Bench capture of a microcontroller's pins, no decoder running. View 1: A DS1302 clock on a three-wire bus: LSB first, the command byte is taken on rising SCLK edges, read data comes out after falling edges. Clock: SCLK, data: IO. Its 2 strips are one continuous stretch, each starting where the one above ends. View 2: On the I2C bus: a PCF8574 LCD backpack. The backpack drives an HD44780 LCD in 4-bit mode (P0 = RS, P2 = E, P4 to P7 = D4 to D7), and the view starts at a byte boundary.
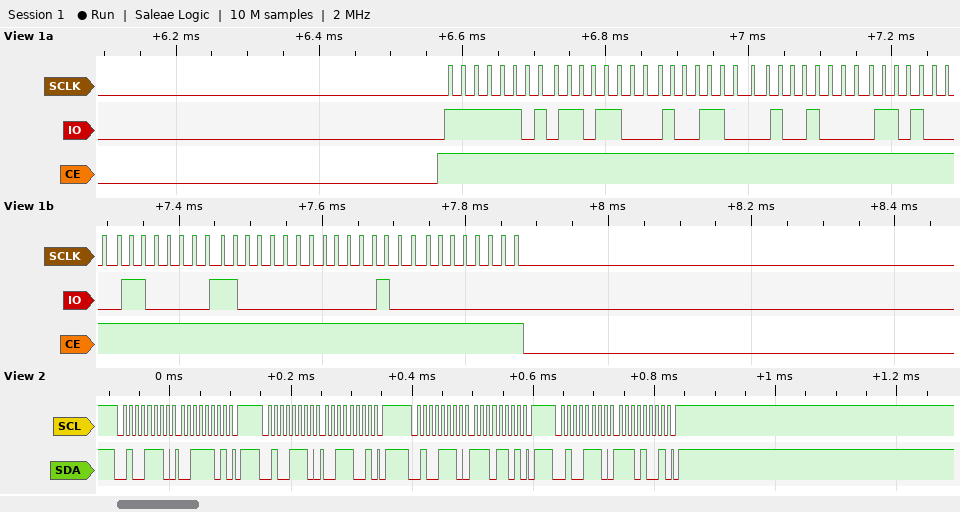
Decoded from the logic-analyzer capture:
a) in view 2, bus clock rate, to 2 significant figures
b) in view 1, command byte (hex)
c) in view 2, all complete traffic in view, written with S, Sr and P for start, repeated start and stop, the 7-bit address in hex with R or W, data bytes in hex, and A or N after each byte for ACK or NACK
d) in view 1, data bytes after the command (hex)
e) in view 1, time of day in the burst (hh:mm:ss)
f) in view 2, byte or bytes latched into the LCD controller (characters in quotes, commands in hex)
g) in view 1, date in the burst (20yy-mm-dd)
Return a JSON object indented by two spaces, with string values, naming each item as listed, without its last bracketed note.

{
  "in view 2, bus clock rate, to 2 significant figures": "100 kHz",
  "in view 1, command byte": "0xBF",
  "in view 2, all complete traffic in view, written with S, Sr and P for start, repeated start and stop, the 7-bit address in hex with R or W, data bytes in hex, and A or N after each byte for ACK or NACK": "S 27W A 3D A P S 27W A 39 A P S 27W A ED A P S 27W A E9 A P",
  "in view 1, data bytes after the command": "36 32 12 16 06 03 20 00",
  "in view 1, time of day in the burst": "12:32:36",
  "in view 2, byte or bytes latched into the LCD controller": "'>'",
  "in view 1, date in the burst": "2020-06-16"
}
